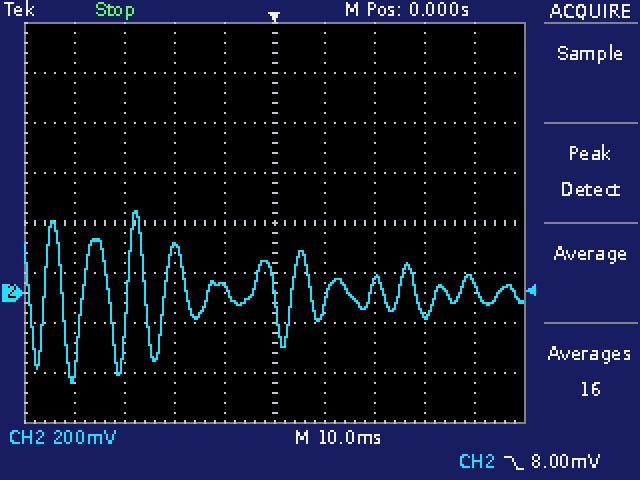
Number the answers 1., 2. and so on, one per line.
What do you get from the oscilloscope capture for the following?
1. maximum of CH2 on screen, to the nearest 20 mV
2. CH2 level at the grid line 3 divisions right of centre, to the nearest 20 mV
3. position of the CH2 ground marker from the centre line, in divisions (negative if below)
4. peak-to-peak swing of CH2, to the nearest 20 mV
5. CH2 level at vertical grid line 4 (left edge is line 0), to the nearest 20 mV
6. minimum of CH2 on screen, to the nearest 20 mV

1. 320 mV
2. -80 mV
3. -1.4 div
4. 680 mV
5. 20 mV
6. -360 mV
